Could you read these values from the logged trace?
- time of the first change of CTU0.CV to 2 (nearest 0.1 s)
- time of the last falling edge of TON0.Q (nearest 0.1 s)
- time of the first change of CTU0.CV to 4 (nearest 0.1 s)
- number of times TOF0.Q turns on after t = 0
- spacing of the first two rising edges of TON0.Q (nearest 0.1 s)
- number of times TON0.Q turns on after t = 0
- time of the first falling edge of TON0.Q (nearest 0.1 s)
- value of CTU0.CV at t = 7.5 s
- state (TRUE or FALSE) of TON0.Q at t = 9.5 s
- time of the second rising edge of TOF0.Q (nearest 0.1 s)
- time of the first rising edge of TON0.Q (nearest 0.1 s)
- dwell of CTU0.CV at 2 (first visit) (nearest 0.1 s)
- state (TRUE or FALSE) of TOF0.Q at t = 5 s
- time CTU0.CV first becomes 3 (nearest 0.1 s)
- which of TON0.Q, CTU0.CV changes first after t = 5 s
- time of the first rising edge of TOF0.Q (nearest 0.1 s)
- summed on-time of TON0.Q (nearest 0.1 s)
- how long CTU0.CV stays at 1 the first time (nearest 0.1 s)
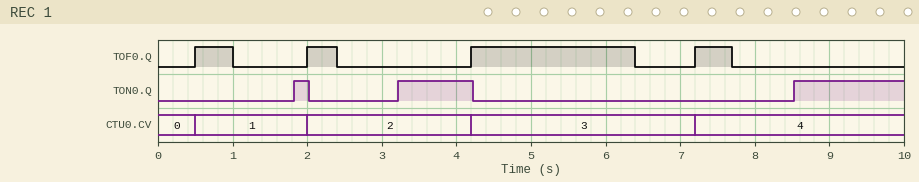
2.0 s
4.2 s
7.2 s
4
1.4 s
3
2.0 s
4
TRUE
2.0 s
1.8 s
2.2 s
TRUE
4.2 s
CTU0.CV
0.5 s
2.7 s
1.5 s
